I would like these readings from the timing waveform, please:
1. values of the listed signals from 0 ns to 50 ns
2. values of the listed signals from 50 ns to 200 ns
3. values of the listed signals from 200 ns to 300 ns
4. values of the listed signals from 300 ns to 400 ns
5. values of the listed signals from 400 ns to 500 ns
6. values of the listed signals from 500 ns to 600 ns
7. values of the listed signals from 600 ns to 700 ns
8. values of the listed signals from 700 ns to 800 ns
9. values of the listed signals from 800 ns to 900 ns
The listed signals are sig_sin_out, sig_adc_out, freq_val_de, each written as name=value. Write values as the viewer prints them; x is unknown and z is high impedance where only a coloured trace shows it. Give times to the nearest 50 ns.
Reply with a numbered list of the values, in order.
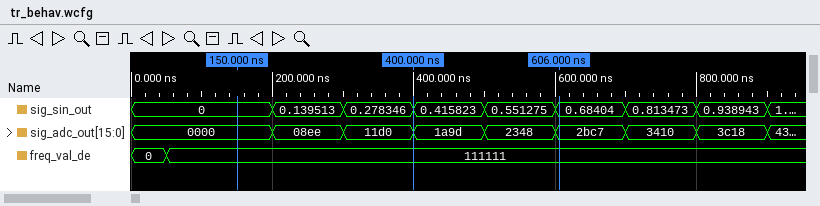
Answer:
1. sig_sin_out=0, sig_adc_out=0000, freq_val_de=0
2. sig_sin_out=0, sig_adc_out=0000, freq_val_de=111111
3. sig_sin_out=0.139513, sig_adc_out=08ee, freq_val_de=111111
4. sig_sin_out=0.278346, sig_adc_out=11d0, freq_val_de=111111
5. sig_sin_out=0.415823, sig_adc_out=1a9d, freq_val_de=111111
6. sig_sin_out=0.551275, sig_adc_out=2348, freq_val_de=111111
7. sig_sin_out=0.68404, sig_adc_out=2bc7, freq_val_de=111111
8. sig_sin_out=0.813473, sig_adc_out=3410, freq_val_de=111111
9. sig_sin_out=0.938943, sig_adc_out=3c18, freq_val_de=111111
